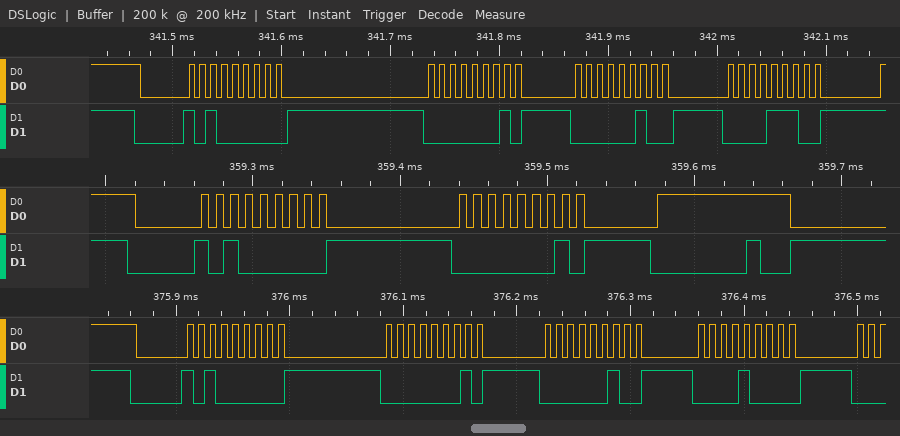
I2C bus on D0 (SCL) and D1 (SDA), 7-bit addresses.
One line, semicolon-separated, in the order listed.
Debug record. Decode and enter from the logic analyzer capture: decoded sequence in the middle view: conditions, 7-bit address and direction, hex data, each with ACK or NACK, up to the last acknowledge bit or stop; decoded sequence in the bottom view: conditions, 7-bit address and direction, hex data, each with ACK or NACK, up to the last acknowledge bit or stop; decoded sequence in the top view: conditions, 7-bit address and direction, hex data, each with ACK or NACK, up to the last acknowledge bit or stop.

start, address 50 write ACK, 01 ACK, stop; start, address 50 write ACK, 01 ACK, 02 ACK, 08 ACK; start, address 50 write ACK, 01 ACK, 02 ACK, 0E ACK
